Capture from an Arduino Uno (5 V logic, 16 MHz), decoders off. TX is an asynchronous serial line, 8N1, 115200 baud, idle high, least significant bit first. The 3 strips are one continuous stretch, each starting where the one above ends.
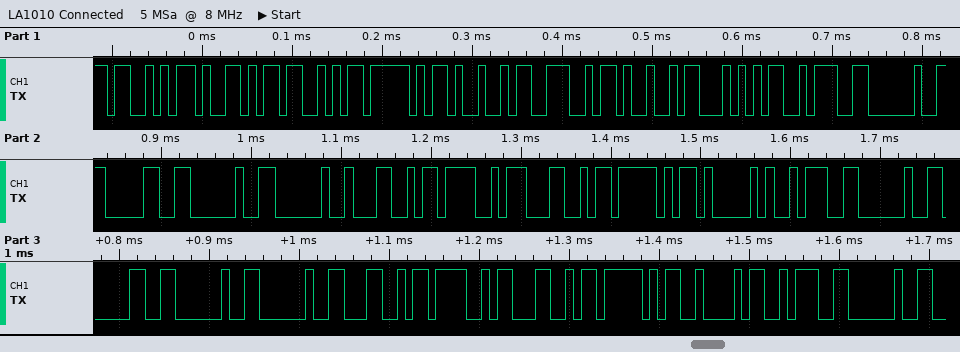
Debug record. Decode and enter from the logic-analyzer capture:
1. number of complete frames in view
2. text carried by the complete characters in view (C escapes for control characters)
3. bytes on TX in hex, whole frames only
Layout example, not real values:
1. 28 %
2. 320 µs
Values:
1. 30
2. "SYS_INIT: 0  LOL_A: 0  LOL_B: "
3. 0x53 0x59 0x53 0x5F 0x49 0x4E 0x49 0x54 0x3A 0x20 0x30 0x20 0x20 0x4C 0x4F 0x4C 0x5F 0x41 0x3A 0x20 0x30 0x20 0x20 0x4C 0x4F 0x4C 0x5F 0x42 0x3A 0x20
